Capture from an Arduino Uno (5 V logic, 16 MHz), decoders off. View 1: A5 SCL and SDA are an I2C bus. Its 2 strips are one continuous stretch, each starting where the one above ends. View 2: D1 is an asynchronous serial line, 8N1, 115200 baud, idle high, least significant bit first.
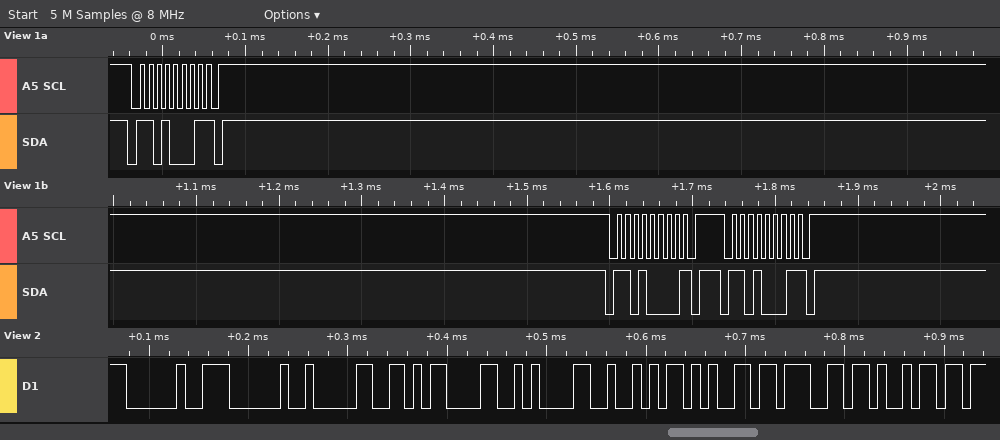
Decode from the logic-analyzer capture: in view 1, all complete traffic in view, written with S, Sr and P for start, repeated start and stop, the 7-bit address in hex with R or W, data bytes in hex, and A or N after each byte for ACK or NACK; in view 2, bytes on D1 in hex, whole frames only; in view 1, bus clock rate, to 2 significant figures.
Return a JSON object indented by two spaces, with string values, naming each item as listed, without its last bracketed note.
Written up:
{
  "in view 1, all complete traffic in view, written with S, Sr and P for start, repeated start and stop, the 7-bit address in hex with R or W, data bytes in hex, and A or N after each byte for ACK or NACK": "S 68R N P S 68W N P S 68R N P",
  "in view 2, bytes on D1 in hex, whole frames only": "20 20 30 0D 0A 52 65 67 69",
  "in view 1, bus clock rate, to 2 significant figures": "100 kHz"
}
